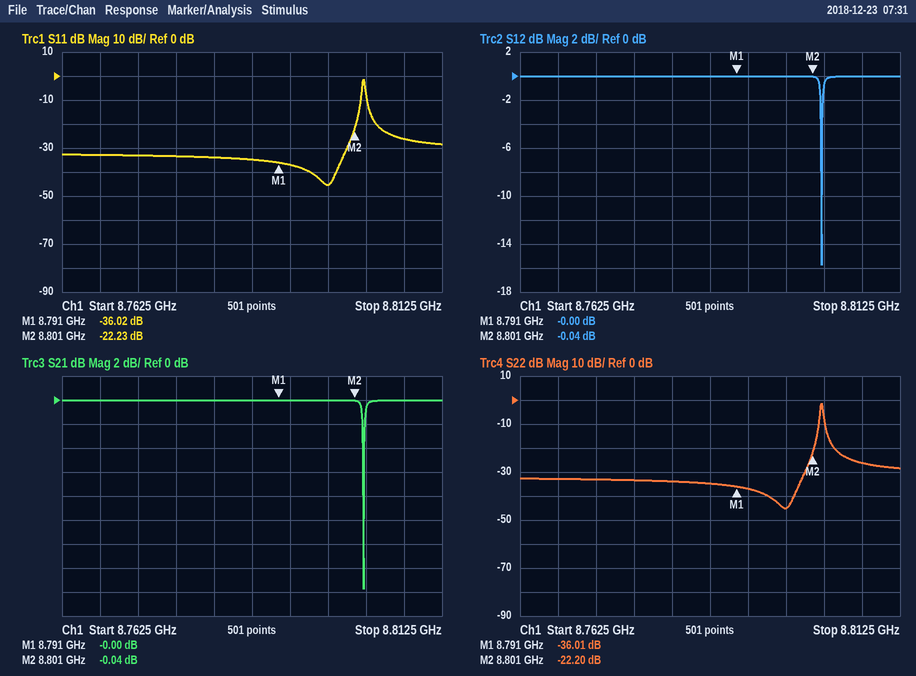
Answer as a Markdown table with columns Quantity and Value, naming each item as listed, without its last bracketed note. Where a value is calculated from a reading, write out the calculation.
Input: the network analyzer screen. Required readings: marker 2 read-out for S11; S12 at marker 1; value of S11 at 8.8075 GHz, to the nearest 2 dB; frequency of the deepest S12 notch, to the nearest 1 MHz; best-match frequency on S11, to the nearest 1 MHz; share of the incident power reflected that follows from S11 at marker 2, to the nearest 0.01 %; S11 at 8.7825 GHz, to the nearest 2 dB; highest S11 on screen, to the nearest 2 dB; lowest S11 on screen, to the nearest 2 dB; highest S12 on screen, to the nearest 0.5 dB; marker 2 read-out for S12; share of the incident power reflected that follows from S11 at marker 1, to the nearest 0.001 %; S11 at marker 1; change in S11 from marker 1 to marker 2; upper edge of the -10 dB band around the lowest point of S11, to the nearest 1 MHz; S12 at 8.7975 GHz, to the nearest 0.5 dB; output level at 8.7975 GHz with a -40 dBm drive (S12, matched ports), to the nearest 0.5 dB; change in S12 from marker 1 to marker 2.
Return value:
| Quantity | Value |
|---|---|
| marker 2 read-out for S11 | -22.23 dB |
| S12 at marker 1 | -0.00 dB |
| value of S11 at 8.8075 GHz, to the nearest 2 dB | -26 dB |
| frequency of the deepest S12 notch, to the nearest 1 MHz | 8.802 GHz |
| best-match frequency on S11, to the nearest 1 MHz | 8.797 GHz |
| share of the incident power reflected that follows from S11 at marker 2, to the nearest 0.01 % | 10^(-22.23/10) ≈ 0.60 % |
| S11 at 8.7825 GHz, to the nearest 2 dB | -34 dB |
| highest S11 on screen, to the nearest 2 dB | -2 dB |
| lowest S11 on screen, to the nearest 2 dB | -46 dB |
| highest S12 on screen, to the nearest 0.5 dB | 0.0 dB |
| marker 2 read-out for S12 | -0.04 dB |
| share of the incident power reflected that follows from S11 at marker 1, to the nearest 0.001 % | 10^(-36.02/10) ≈ 0.025 % |
| S11 at marker 1 | -36.02 dB |
| change in S11 from marker 1 to marker 2 | -22.23 − (-36.02) = 13.79 dB |
| upper edge of the -10 dB band around the lowest point of S11, to the nearest 1 MHz | 8.802 GHz |
| S12 at 8.7975 GHz, to the nearest 0.5 dB | 0.0 dB |
| output level at 8.7975 GHz with a -40 dBm drive (S12, matched ports), to the nearest 0.5 dB | -40 dBm + (0.0 dB) = -40.0 dBm |
| change in S12 from marker 1 to marker 2 | -0.04 − (-0) = -0.04 dB |
